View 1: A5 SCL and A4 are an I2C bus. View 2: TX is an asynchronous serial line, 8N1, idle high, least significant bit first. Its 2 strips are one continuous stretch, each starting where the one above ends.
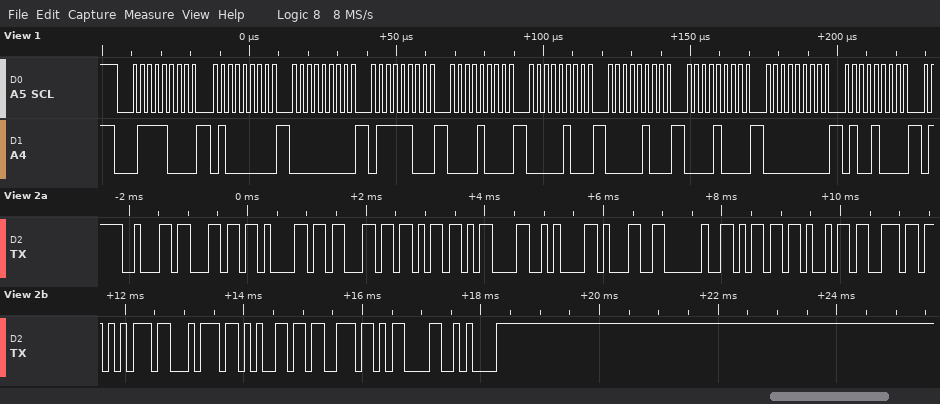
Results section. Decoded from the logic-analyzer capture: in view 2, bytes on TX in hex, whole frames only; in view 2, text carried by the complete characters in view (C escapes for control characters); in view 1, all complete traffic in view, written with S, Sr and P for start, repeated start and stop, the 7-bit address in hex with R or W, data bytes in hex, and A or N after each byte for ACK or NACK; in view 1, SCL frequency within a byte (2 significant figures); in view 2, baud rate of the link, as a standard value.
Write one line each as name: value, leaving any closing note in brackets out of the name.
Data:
in view 2, bytes on TX in hex, whole frames only: 62 6C 61 63 6B 0D 0A 31 20 6D 69 6E 75 74 65 73 0D 0A
in view 2, text carried by the complete characters in view: "black\r\n1 minutes\r\n"
in view 1, all complete traffic in view, written with S, Sr and P for start, repeated start and stop, the 7-bit address in hex with R or W, data bytes in hex, and A or N after each byte for ACK or NACK: S 3CW A 40 A 00 A 7C A 08 A 04 A 04 A 08 A 00 A 48 A
in view 1, SCL frequency within a byte: 400 kHz
in view 2, baud rate of the link, as a standard value: 9600 baud
